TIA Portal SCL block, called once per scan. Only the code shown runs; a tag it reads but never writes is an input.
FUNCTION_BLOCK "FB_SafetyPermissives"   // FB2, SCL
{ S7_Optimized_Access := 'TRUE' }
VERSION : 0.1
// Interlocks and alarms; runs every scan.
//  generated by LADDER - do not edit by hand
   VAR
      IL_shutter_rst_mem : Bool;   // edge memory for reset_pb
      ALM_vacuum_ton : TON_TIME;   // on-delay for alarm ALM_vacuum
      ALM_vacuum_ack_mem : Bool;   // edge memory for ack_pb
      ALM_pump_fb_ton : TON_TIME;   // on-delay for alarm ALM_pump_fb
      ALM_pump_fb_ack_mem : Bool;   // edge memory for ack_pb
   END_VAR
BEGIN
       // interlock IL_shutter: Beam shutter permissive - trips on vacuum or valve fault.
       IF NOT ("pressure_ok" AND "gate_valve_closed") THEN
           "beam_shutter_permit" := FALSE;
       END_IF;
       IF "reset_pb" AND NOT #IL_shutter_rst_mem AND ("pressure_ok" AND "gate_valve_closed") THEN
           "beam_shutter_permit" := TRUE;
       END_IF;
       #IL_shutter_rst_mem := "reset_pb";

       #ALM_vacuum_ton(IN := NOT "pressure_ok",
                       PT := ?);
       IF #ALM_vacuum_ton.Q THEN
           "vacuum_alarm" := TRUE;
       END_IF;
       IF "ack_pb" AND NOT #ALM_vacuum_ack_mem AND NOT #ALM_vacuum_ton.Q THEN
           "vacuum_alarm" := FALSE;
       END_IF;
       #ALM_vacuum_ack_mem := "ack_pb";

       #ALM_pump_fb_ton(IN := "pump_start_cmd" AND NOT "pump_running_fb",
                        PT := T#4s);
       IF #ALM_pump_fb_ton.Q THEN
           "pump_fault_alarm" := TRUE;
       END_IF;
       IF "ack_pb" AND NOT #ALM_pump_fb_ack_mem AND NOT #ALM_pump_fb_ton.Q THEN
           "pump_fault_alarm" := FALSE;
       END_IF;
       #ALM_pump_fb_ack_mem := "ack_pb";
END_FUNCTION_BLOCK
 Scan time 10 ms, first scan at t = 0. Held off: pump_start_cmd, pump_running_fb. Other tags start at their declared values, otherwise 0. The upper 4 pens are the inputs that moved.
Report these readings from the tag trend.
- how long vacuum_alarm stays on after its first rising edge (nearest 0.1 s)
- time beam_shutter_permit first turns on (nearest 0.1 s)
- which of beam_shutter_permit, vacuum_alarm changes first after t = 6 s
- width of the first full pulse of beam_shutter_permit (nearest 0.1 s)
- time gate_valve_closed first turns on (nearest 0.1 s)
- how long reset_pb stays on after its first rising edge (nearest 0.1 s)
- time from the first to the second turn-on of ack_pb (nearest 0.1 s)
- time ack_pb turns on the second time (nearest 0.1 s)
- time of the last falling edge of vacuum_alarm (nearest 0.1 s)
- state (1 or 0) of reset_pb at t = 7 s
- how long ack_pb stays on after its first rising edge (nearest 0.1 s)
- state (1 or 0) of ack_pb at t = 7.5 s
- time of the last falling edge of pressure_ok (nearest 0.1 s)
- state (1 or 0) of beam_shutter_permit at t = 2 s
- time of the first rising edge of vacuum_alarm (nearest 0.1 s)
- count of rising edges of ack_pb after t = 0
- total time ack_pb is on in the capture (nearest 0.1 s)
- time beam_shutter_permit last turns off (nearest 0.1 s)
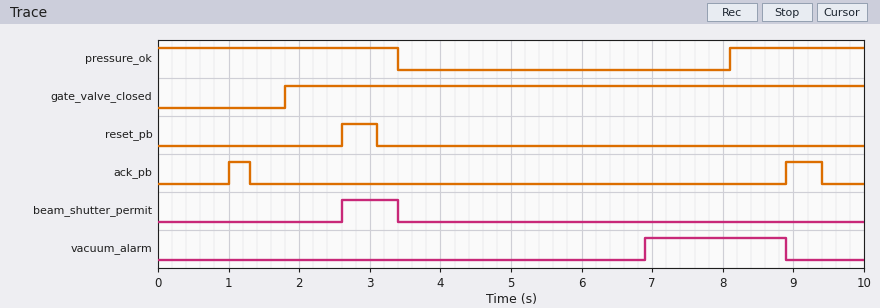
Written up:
2.0 s
2.6 s
vacuum_alarm
0.8 s
1.8 s
0.5 s
7.9 s
8.9 s
8.9 s
0
0.3 s
0
3.4 s
0
6.9 s
2
0.8 s
3.4 s
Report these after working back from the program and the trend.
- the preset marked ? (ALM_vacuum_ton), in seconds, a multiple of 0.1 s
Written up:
3.5 s
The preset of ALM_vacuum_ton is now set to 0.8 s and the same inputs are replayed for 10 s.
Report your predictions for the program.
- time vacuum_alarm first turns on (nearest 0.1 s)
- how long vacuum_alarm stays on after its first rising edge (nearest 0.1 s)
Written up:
4.2 s
4.7 s
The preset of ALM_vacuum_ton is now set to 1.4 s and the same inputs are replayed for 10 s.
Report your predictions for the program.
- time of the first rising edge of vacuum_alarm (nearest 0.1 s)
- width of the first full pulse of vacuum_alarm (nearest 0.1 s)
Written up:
4.8 s
4.1 s
